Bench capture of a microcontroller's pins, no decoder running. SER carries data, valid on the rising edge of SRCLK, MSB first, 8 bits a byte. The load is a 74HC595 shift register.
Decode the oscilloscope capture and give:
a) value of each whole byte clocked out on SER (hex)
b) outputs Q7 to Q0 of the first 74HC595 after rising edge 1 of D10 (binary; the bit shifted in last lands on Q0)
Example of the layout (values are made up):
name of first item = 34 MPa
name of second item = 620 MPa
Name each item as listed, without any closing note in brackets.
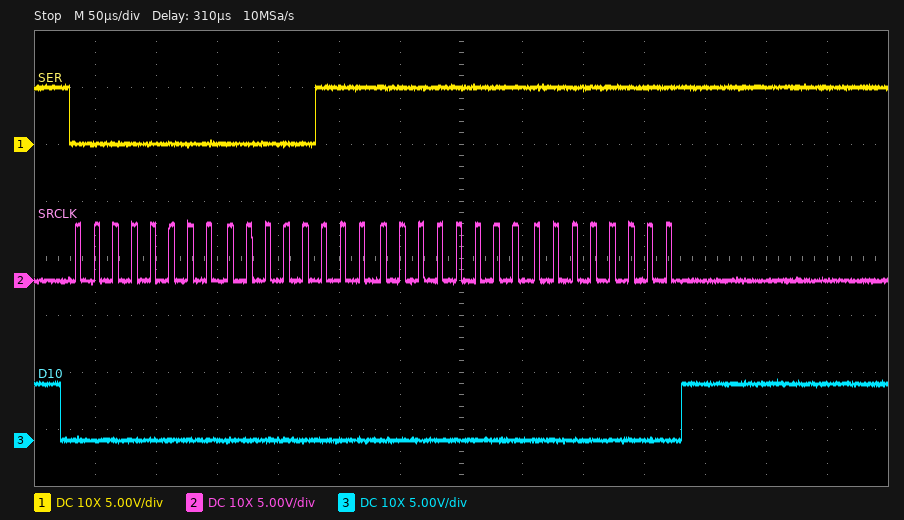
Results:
value of each whole byte clocked out on SER = 0x00 0x07 0xFF 0xFF
outputs Q7 to Q0 of the first 74HC595 after rising edge 1 of D10 = 11111111
